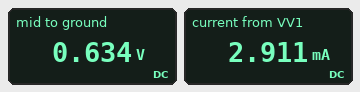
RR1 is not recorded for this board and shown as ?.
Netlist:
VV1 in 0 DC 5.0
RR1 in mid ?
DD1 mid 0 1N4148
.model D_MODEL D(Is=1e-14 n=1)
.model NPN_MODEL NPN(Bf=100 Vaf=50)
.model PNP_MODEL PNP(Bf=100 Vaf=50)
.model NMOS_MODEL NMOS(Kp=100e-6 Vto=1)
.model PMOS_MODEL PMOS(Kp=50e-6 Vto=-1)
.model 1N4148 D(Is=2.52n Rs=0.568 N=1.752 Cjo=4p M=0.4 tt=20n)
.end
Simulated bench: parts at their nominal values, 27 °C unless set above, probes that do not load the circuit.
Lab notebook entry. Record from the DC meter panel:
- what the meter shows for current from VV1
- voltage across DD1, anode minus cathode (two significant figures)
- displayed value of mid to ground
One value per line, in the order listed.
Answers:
2.911 mA
630 mV
0.634 V
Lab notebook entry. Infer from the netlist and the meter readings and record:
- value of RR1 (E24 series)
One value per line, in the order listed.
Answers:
1.5 kΩ
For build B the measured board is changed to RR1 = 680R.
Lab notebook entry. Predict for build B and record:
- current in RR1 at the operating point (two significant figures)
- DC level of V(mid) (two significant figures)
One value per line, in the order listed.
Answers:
6.4 mA
670 mV
